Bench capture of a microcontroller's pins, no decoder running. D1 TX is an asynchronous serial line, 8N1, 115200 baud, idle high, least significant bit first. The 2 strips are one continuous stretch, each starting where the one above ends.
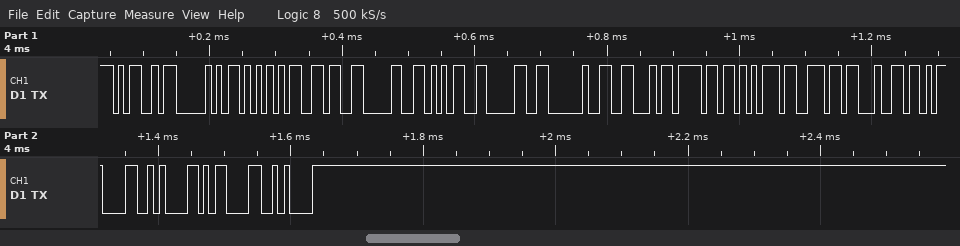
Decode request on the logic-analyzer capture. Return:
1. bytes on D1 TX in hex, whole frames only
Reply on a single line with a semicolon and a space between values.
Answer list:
0x4D 0x50 0x55 0x36 0x30 0x35 0x30 0x20 0x46 0x6F 0x75 0x6E 0x64 0x0D 0x0A 0x0D 0x0A
